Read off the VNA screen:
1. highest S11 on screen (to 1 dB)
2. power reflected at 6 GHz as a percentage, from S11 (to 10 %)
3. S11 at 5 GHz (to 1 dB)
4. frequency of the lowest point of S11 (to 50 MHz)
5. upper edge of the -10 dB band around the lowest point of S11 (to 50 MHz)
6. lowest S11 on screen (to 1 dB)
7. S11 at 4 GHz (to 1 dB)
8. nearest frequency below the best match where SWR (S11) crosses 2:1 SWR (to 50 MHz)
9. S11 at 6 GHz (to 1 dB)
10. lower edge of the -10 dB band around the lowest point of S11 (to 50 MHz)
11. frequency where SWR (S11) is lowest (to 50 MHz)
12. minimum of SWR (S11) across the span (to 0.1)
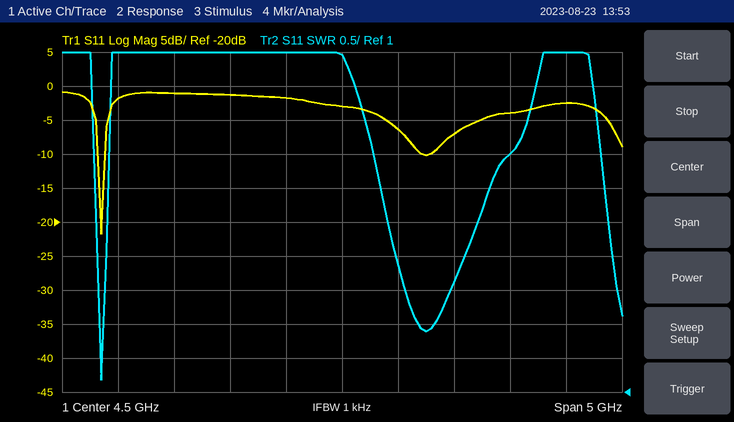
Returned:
-1 dB
40 %
-6 dB
2.35 GHz
2.40 GHz
-22 dB
-2 dB
2.35 GHz
-4 dB
2.30 GHz
2.35 GHz
1.2
